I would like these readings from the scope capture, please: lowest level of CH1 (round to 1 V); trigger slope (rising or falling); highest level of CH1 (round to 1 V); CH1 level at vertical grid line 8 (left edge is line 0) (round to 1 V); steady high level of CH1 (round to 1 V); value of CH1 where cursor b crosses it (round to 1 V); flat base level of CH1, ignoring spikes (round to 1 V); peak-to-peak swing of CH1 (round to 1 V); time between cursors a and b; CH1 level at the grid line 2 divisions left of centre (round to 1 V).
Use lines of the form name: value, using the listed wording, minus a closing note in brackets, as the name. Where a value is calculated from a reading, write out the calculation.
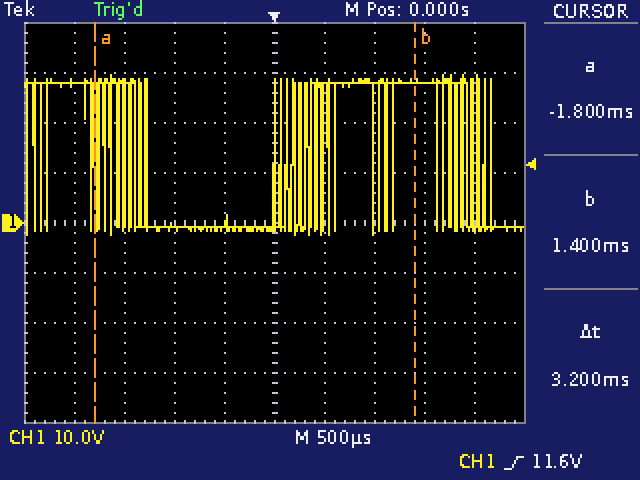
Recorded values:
lowest level of CH1: -2 V
trigger slope: rising
highest level of CH1: 30 V
CH1 level at vertical grid line 8 (left edge is line 0): 28 V
steady high level of CH1: 28 V
value of CH1 where cursor b crosses it: 28 V
flat base level of CH1, ignoring spikes: -1 V
peak-to-peak swing of CH1: 30 V − (-2 V) = 32 V
time between cursors a and b: 3.2 ms
CH1 level at the grid line 2 divisions left of centre: -1 V
